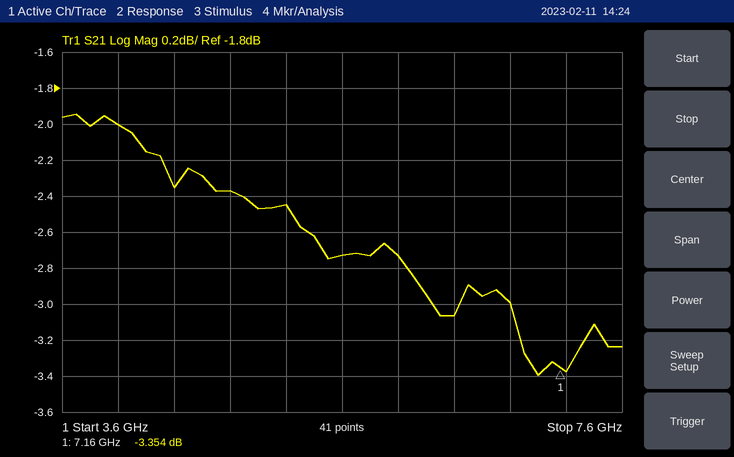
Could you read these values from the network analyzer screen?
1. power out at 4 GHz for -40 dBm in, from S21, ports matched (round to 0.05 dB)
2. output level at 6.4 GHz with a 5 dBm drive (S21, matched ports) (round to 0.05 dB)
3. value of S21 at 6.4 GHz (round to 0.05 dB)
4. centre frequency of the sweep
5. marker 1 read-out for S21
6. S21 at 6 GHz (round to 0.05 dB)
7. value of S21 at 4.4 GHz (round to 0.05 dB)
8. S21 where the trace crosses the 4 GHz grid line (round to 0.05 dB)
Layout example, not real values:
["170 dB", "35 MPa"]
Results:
["-42.00 dBm", "1.95 dBm", "-3.05 dB", "5.6 GHz", "-3.354 dB", "-2.75 dB", "-2.35 dB", "-2.00 dB"]
